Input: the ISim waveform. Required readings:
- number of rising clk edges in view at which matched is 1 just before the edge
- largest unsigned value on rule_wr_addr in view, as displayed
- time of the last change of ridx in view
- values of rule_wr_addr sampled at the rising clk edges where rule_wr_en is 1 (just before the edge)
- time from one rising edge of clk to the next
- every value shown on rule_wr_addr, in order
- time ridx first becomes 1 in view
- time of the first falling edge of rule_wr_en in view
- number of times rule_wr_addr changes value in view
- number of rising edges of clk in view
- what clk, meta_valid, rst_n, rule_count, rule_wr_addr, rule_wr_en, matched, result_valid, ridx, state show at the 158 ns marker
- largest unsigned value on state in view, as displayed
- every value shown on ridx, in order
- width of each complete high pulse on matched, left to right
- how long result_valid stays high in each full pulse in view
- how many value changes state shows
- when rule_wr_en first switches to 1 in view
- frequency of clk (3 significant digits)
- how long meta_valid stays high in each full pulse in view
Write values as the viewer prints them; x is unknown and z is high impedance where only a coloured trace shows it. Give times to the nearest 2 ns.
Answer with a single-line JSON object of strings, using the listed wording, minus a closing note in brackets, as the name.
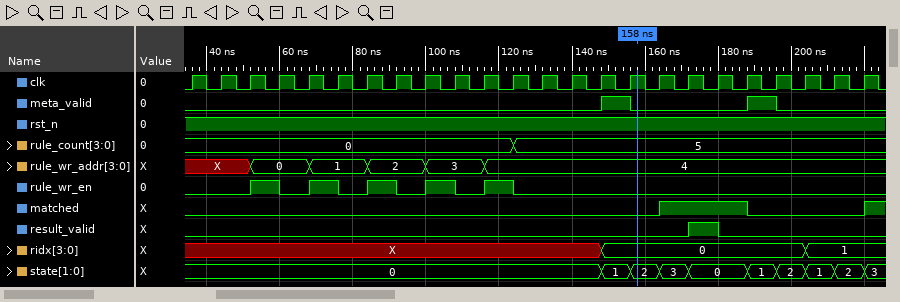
{"number of rising clk edges in view at which matched is 1 just before the edge": "3", "largest unsigned value on rule_wr_addr in view, as displayed": "4", "time of the last change of ridx in view": "204 ns", "values of rule_wr_addr sampled at the rising clk edges where rule_wr_en is 1": "0, 1, 2, 3, 4", "time from one rising edge of clk to the next": "8 ns", "every value shown on rule_wr_addr, in order": "X, 0, 1, 2, 3, 4", "time ridx first becomes 1 in view": "204 ns", "time of the first falling edge of rule_wr_en in view": "60 ns", "number of times rule_wr_addr changes value in view": "5", "number of rising edges of clk in view": "24", "what clk, meta_valid, rst_n, rule_count, rule_wr_addr, rule_wr_en, matched, result_valid, ridx, state show at the 158 ns marker": "clk=1, meta_valid=0, rst_n=1, rule_count=5, rule_wr_addr=4, rule_wr_en=0, matched=0, result_valid=0, ridx=0, state=2", "largest unsigned value on state in view, as displayed": "3", "every value shown on ridx, in order": "X, 0, 1", "width of each complete high pulse on matched, left to right": "24 ns", "how long result_valid stays high in each full pulse in view": "8 ns", "how many value changes state shows": "9", "when rule_wr_en first switches to 1 in view": "52 ns", "frequency of clk": "125 MHz", "how long meta_valid stays high in each full pulse in view": "8 ns, 8 ns"}
